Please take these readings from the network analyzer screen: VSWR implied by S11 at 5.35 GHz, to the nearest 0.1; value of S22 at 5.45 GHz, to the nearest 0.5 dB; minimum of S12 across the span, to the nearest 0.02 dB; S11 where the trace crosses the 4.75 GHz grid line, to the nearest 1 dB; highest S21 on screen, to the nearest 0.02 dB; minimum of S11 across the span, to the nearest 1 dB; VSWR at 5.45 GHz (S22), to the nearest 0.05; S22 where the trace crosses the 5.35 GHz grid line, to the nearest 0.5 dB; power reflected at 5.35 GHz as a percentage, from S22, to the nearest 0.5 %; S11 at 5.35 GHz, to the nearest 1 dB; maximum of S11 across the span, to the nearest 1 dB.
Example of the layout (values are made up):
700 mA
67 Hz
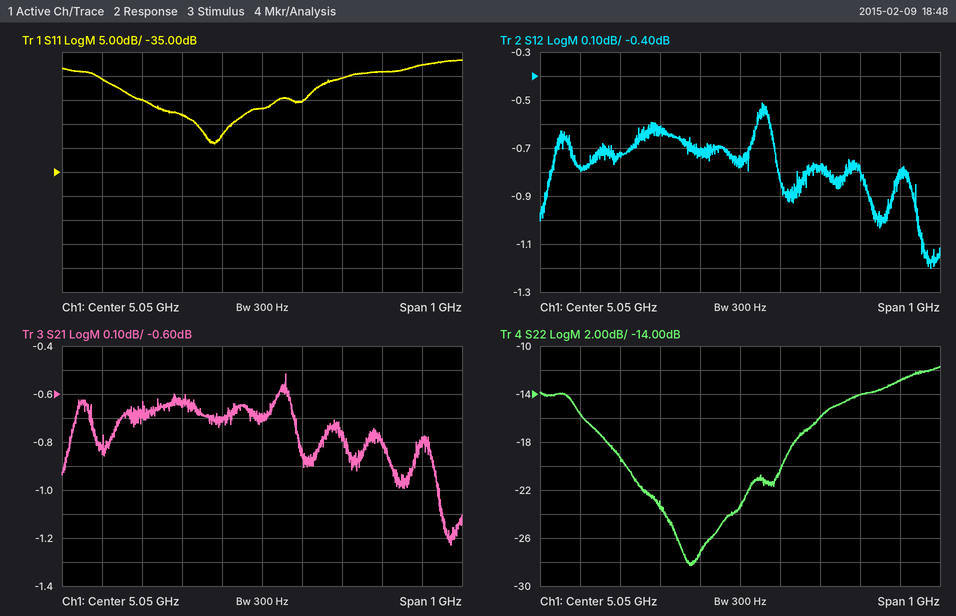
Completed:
1.5
-13.0 dB
-1.20 dB
-20 dB
-0.52 dB
-29 dB
1.60
-14.0 dB
4.0 %
-14 dB
-12 dB
